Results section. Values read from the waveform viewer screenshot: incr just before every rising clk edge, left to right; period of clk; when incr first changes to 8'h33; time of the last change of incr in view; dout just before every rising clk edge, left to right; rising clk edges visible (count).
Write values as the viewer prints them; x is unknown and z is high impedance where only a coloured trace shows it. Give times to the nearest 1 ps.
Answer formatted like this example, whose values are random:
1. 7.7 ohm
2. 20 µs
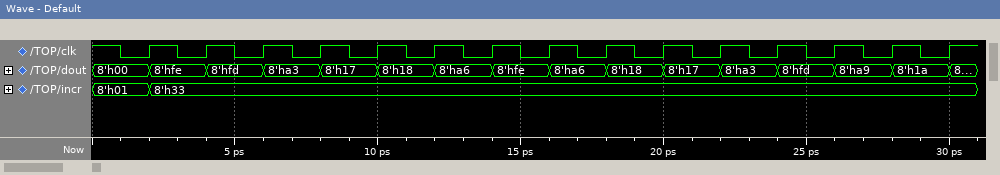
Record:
1. 8'h01, 8'h33, 8'h33, 8'h33, 8'h33, 8'h33, 8'h33, 8'h33, 8'h33, 8'h33, 8'h33, 8'h33, 8'h33, 8'h33, 8'h33
2. 2 ps
3. 2 ps
4. 2 ps
5. 8'h00, 8'hfe, 8'hfd, 8'ha3, 8'h17, 8'h18, 8'ha6, 8'hfe, 8'ha6, 8'h18, 8'h17, 8'ha3, 8'hfd, 8'ha9, 8'h1a
6. 15
